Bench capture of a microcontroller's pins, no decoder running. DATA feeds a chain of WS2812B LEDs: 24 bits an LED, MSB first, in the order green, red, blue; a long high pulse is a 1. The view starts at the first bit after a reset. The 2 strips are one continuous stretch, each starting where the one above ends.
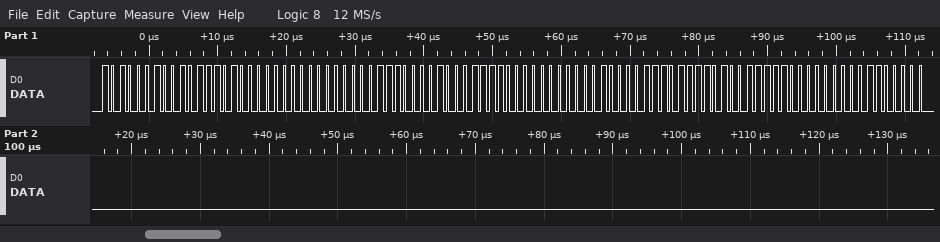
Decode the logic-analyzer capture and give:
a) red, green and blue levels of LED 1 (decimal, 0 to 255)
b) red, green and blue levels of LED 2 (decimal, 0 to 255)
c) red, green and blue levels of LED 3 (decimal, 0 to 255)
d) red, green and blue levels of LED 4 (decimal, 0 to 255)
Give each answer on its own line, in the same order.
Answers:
93, 162, 0
225, 0, 30
33, 0, 222
0, 159, 96
